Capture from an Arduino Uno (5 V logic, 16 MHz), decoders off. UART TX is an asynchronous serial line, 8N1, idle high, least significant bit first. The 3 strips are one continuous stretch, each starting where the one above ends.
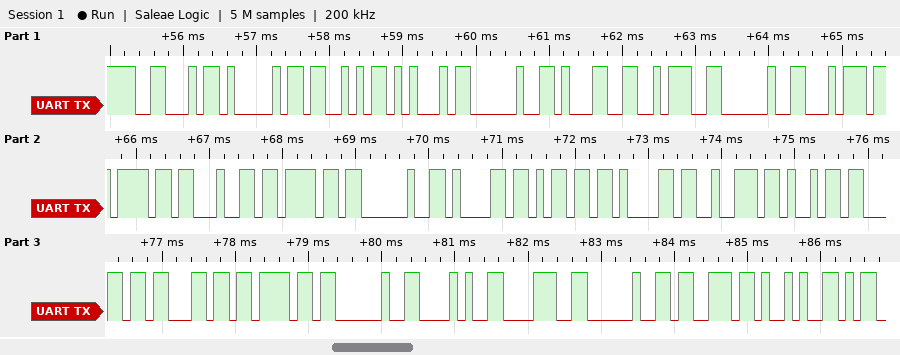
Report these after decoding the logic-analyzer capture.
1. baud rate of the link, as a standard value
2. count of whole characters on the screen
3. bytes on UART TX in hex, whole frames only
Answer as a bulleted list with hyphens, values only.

- 9600 baud
- 27
- 46 41 53 45 20 31 3A 20 74 6F 64 6F 20 61 6D 61 72 69 6C 6C 6F 20 28 38 20 73 29
